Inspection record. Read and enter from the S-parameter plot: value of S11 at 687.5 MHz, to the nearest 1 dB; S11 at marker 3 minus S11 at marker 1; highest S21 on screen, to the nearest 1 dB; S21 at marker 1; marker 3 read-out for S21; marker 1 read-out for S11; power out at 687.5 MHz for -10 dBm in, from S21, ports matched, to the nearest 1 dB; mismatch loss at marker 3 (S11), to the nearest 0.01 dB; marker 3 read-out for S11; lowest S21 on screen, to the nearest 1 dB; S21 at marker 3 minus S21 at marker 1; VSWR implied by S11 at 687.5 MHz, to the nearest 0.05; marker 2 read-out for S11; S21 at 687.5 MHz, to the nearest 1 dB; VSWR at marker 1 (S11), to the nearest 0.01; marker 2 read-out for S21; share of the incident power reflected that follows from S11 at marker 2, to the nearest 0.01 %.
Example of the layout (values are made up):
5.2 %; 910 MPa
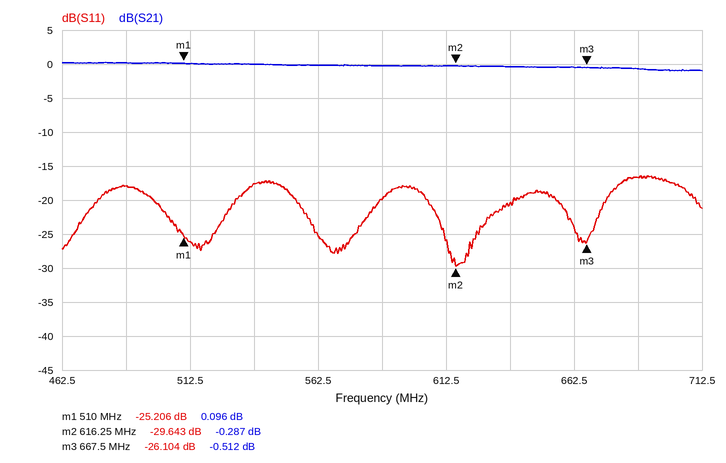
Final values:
-17 dB; -0.898 dB; 0 dB; 0.096 dB; -0.512 dB; -25.206 dB; -11 dBm; 0.01 dB; -26.104 dB; -1 dB; -0.608 dB; 1.35; -29.643 dB; -1 dB; 1.12; -0.287 dB; 0.11 %
